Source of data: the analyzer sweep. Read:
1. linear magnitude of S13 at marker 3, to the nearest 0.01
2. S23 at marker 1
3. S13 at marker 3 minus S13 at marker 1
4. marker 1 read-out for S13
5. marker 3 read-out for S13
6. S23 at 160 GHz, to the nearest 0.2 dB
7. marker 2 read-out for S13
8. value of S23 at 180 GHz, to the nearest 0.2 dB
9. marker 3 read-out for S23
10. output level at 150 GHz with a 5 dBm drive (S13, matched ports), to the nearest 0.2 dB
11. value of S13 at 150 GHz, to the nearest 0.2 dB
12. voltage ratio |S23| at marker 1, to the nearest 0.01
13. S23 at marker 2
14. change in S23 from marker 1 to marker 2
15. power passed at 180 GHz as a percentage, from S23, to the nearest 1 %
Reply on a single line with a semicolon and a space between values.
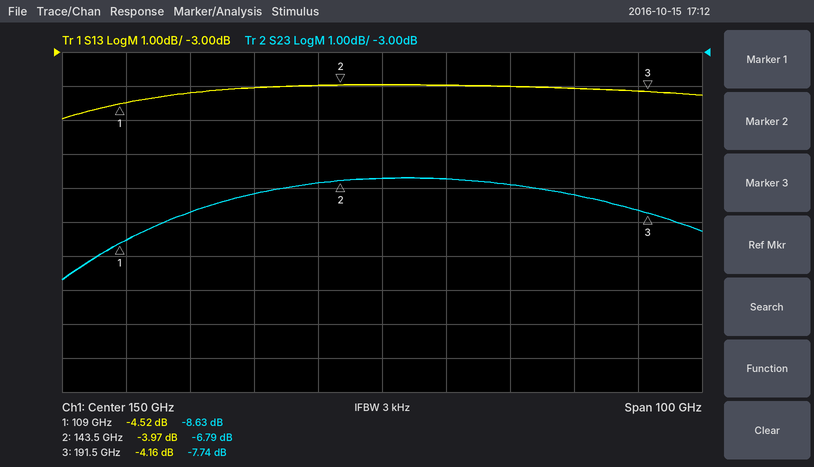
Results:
0.62; -8.63 dB; 0.36 dB; -4.52 dB; -4.16 dB; -6.8 dB; -3.97 dB; -7.2 dB; -7.74 dB; 1.0 dBm; -4.0 dB; 0.37; -6.79 dB; 1.84 dB; 19 %
